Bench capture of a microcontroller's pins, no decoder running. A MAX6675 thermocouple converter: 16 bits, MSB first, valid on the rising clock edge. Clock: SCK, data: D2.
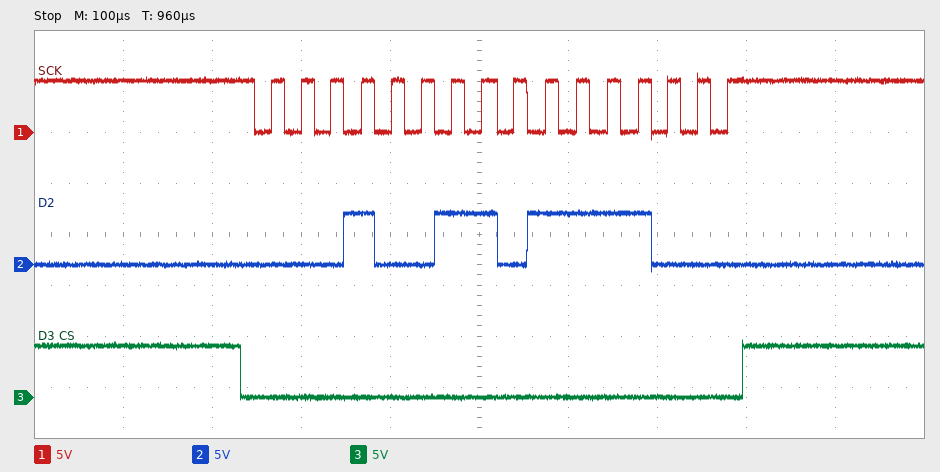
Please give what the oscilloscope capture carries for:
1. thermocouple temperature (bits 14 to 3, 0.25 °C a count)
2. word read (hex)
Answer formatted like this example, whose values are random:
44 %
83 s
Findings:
155.75 °C
0x1378
